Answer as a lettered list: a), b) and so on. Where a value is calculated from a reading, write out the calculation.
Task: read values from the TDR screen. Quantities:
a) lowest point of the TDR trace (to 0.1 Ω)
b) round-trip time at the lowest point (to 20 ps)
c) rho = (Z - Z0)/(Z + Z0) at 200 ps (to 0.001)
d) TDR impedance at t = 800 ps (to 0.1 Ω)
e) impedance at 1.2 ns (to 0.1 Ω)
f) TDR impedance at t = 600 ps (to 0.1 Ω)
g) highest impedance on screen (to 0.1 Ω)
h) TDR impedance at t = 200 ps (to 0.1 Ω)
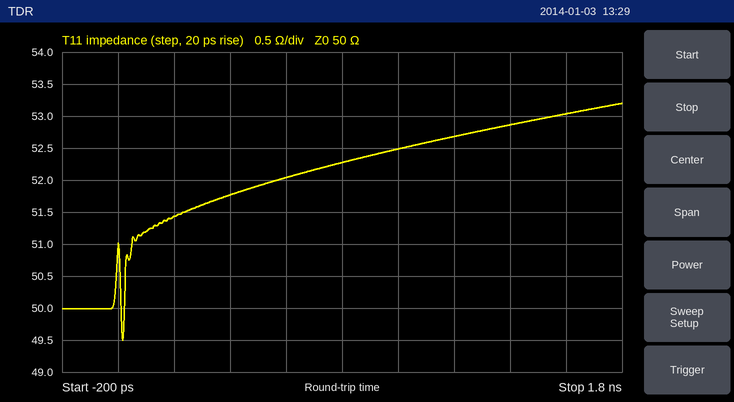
a) 49.5 Ω
b) 20 ps
c) (51.4 − 50)/(51.4 + 50) ≈ +0.014
d) 52.3 Ω
e) 52.7 Ω
f) 52.0 Ω
g) 53.2 Ω
h) 51.4 Ω
